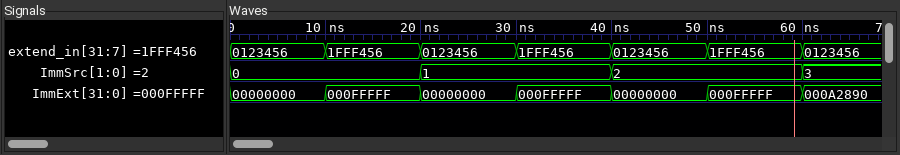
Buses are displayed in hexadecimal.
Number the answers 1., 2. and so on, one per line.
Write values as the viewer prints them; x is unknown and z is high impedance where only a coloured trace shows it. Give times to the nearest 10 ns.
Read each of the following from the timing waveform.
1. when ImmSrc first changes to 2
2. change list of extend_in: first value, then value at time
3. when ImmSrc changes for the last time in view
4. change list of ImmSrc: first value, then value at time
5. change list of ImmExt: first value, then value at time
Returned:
1. 40 ns
2. 0123456, 1FFF456 at 10 ns, 0123456 at 20 ns, 1FFF456 at 30 ns, 0123456 at 40 ns, 1FFF456 at 50 ns, 0123456 at 60 ns
3. 60 ns
4. 0, 1 at 20 ns, 2 at 40 ns, 3 at 60 ns
5. 00000000, 000FFFFF at 10 ns, 00000000 at 20 ns, 000FFFFF at 30 ns, 00000000 at 40 ns, 000FFFFF at 50 ns, 000A2890 at 60 ns
